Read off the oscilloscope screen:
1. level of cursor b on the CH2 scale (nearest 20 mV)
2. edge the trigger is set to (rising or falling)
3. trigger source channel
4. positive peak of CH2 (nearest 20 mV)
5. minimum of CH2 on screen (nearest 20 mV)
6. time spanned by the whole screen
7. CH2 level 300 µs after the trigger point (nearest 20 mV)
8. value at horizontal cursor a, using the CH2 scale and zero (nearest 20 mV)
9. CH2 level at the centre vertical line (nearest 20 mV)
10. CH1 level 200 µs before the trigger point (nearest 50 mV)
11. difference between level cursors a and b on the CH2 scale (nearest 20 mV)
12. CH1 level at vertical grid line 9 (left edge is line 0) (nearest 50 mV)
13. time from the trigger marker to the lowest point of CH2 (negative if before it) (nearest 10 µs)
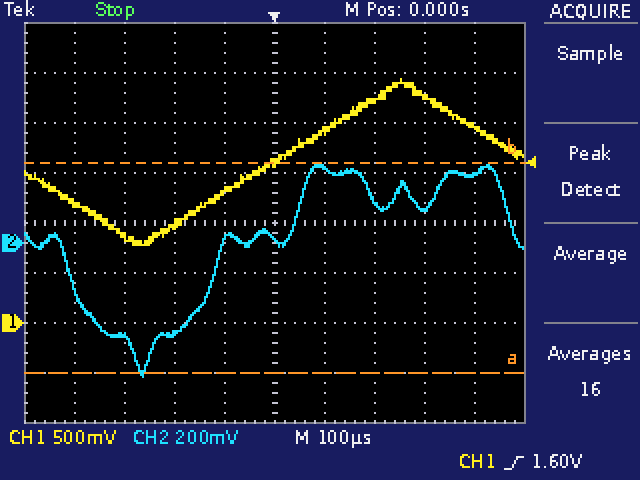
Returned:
320 mV
rising
CH1
320 mV
-540 mV
1 ms
140 mV
-520 mV
20 mV
1.00 V
840 mV
1.95 V
-260 µs
